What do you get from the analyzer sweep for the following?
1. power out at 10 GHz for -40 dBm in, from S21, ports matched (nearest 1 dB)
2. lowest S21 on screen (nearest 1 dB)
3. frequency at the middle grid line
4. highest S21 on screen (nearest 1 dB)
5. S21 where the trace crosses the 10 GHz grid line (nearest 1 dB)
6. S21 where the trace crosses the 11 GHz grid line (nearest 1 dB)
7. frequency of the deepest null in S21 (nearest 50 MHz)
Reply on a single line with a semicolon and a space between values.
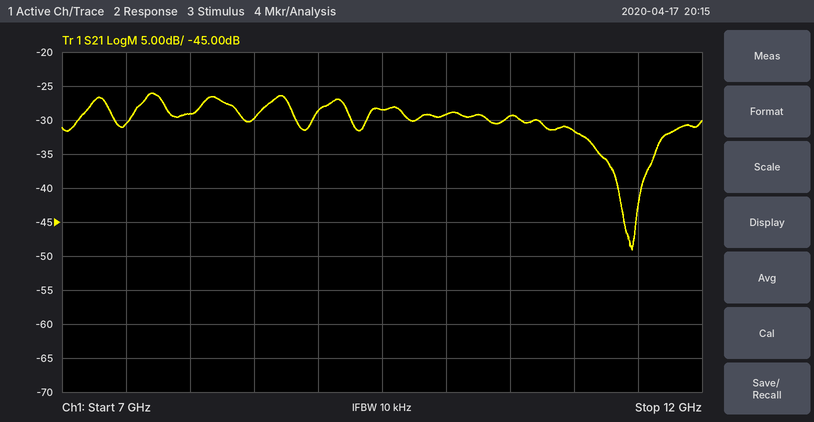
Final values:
-69 dBm; -49 dB; 9.5 GHz; -26 dB; -29 dB; -32 dB; 11.45 GHz
